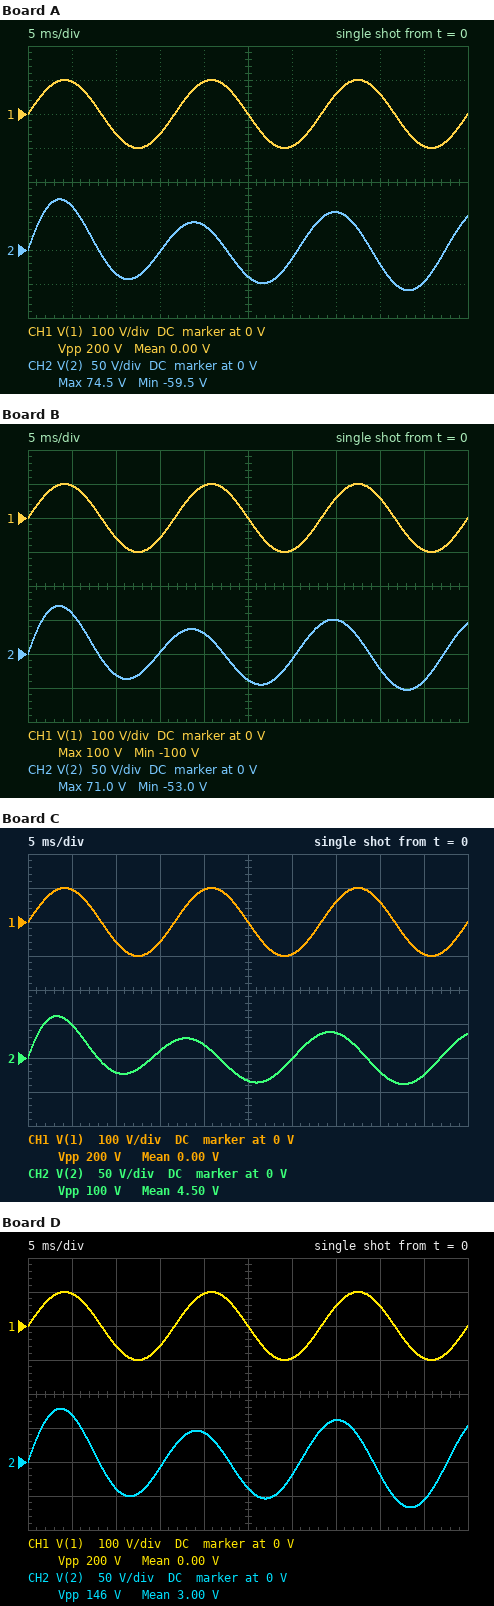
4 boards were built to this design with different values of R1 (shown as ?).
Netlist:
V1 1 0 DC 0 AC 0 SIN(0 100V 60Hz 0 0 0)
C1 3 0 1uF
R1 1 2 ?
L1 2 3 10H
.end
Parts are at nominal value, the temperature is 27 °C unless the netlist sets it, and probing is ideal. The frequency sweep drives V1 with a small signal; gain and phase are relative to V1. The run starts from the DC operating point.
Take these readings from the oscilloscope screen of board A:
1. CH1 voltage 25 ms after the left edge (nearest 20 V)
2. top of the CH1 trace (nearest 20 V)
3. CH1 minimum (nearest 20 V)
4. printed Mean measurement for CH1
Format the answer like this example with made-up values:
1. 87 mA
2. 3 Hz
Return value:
1. 0 V
2. 100 V
3. -100 V
4. 0.00 V
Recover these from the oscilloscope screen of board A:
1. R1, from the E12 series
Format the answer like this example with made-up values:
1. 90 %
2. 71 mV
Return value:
1. 1.5 kΩ
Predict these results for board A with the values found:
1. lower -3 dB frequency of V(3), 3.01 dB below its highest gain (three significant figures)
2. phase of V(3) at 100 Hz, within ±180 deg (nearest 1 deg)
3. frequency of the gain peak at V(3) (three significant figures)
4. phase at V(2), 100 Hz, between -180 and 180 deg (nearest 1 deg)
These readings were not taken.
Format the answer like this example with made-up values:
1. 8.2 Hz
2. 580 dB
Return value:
1. 32.9 Hz
2. -162 deg
3. 47.4 Hz
4. 18 deg
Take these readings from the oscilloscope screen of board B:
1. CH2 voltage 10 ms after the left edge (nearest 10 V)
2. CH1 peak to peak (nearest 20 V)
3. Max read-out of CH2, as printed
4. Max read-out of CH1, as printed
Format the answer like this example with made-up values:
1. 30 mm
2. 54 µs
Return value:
1. -30 V
2. 200 V
3. 71.0 V
4. 100 V
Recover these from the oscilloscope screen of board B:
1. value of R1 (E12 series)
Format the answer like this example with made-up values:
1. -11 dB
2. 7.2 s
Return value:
1. 1.8 kΩ
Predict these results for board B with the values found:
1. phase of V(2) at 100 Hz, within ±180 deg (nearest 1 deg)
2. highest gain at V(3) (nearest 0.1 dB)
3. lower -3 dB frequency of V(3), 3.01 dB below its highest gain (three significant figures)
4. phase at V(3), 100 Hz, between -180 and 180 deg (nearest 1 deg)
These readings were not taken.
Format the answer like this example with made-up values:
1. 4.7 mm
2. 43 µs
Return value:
1. 21 deg
2. 5.3 dB
3. 27.2 Hz
4. -159 deg
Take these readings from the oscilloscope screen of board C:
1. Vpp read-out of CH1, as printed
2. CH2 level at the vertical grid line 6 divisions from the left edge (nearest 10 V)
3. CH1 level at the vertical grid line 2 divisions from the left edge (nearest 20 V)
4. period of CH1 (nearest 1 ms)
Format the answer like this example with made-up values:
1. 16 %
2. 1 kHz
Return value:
1. 200 V
2. 0 V
3. -60 V
4. 17 ms
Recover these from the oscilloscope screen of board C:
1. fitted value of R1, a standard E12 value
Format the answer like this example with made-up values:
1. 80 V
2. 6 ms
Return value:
1. 2.7 kΩ
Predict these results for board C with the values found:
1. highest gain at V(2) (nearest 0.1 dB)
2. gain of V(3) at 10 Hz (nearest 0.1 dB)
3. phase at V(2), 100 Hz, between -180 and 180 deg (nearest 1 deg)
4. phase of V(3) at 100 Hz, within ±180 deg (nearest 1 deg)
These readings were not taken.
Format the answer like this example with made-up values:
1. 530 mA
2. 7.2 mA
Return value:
1. 0 dB
2. 0.2 dB
3. 30 deg
4. -150 deg
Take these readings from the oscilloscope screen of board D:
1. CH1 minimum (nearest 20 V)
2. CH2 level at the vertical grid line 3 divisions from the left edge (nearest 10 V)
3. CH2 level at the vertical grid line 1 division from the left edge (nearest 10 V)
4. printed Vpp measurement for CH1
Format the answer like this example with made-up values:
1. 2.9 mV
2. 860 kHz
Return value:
1. -100 V
2. -10 V
3. 70 V
4. 200 V
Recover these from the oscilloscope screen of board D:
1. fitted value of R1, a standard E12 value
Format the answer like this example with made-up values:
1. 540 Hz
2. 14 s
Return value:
1. 1.2 kΩ
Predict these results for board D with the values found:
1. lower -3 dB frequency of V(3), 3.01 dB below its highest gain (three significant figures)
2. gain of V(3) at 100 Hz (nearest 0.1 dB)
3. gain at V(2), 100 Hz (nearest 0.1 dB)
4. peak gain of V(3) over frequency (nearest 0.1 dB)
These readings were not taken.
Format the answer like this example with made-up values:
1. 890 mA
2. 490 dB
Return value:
1. 37.5 Hz
2. -9.7 dB
3. -0.3 dB
4. 8.6 dB
